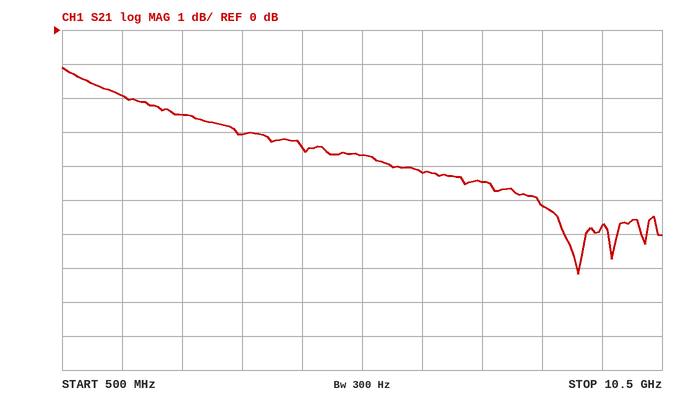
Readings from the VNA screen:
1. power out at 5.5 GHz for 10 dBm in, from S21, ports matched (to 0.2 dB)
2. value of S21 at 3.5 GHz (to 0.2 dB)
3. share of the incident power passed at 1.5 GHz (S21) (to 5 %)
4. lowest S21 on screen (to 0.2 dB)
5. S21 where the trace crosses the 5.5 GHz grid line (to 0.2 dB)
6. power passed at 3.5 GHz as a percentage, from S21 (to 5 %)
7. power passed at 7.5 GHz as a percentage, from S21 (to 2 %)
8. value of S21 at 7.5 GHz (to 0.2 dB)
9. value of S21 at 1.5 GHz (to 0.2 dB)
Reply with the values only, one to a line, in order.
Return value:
6.4 dBm
-3.0 dB
65 %
-7.2 dB
-3.6 dB
50 %
36 %
-4.4 dB
-2.0 dB
